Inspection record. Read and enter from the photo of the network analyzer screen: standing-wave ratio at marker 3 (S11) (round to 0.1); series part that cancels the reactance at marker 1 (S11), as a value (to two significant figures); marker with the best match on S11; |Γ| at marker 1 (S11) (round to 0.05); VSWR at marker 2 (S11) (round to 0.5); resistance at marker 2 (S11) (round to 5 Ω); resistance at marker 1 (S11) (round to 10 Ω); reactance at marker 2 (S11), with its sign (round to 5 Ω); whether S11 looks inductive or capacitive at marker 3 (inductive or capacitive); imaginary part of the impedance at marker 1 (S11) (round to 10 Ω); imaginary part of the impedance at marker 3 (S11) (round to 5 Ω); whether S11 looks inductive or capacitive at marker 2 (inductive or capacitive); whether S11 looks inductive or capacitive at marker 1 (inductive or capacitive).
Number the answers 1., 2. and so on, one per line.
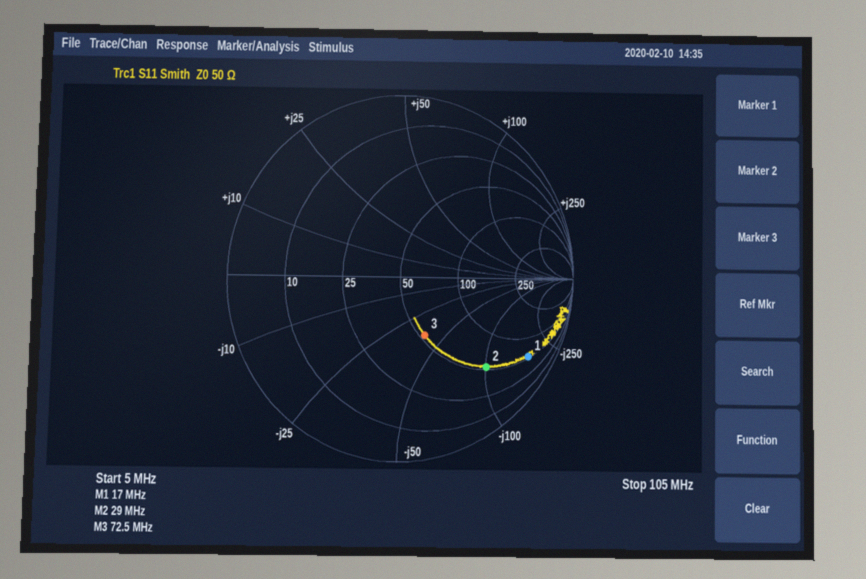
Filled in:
1. 2.1
2. 1.6 µH
3. marker 3
4. 0.85
5. 5.5
6. 55 Ω
7. 50 Ω
8. -100 Ω
9. capacitive
10. -170 Ω
11. -40 Ω
12. capacitive
13. capacitive
